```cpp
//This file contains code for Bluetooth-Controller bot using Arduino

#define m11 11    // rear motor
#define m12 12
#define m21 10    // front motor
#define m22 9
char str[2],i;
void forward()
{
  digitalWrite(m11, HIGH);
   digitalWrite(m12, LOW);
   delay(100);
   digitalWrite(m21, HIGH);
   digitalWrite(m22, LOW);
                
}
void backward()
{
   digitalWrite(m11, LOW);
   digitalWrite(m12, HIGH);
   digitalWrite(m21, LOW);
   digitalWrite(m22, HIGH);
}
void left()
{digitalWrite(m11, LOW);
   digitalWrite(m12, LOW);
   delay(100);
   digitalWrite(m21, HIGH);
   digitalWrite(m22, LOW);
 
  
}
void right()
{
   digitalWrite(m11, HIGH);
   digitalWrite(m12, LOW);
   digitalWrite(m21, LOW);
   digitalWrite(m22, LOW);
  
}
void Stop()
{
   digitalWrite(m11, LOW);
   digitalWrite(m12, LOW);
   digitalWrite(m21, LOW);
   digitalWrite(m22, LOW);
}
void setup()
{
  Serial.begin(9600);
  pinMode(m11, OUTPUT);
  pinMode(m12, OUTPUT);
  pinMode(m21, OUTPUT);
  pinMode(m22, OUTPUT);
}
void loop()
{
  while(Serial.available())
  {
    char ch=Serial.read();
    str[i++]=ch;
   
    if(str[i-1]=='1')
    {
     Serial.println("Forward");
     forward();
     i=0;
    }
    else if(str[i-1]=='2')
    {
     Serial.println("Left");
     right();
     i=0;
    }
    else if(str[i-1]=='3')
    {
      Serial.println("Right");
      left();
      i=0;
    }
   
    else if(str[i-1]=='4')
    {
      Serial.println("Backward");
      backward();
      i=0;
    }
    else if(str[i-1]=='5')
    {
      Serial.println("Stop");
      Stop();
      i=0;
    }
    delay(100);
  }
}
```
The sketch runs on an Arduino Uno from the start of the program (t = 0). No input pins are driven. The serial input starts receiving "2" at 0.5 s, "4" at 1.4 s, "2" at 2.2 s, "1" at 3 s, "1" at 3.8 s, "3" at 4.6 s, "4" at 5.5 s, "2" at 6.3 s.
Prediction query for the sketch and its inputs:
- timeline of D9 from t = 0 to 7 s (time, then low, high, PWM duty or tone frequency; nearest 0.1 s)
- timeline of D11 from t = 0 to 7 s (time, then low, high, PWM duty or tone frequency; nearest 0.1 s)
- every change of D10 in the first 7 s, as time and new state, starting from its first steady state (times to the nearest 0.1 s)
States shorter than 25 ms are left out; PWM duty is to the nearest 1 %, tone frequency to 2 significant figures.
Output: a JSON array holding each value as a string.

["0 s low; 1.4 s high; 2.2 s low; 5.5 s high; 6.3 s low", "0 s low; 0.5 s high; 1.4 s low; 2.2 s high; 4.6 s low; 6.3 s high", "0 s low; 3.1 s high; 5.5 s low"]
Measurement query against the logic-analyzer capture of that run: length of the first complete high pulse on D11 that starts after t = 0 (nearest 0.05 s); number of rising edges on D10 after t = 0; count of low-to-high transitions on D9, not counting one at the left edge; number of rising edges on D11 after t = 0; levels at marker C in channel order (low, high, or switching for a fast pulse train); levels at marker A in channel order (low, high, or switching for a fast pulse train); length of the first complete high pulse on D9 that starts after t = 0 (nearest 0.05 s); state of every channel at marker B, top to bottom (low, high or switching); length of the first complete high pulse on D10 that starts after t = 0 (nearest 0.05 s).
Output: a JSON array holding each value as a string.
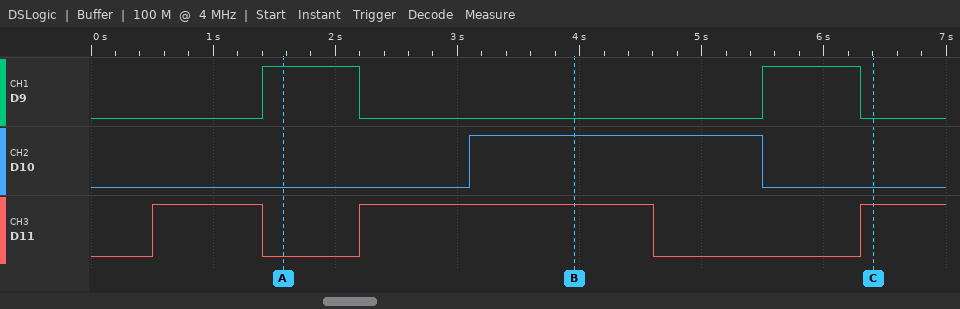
["0.90 s", "1", "2", "3", "D9 low, D10 low, D11 high", "D9 high, D10 low, D11 low", "0.80 s", "D9 low, D10 high, D11 high", "2.40 s"]
